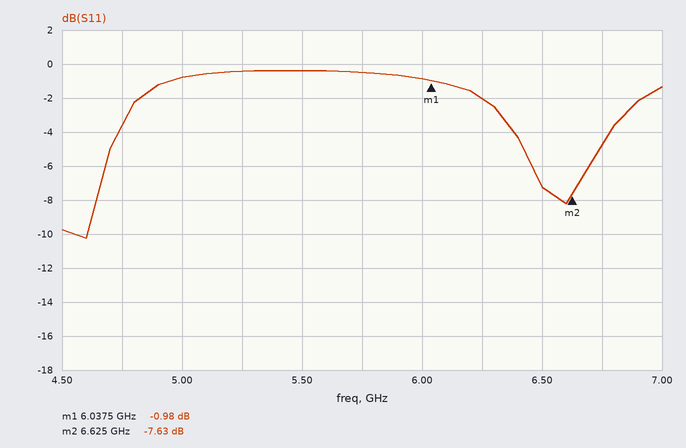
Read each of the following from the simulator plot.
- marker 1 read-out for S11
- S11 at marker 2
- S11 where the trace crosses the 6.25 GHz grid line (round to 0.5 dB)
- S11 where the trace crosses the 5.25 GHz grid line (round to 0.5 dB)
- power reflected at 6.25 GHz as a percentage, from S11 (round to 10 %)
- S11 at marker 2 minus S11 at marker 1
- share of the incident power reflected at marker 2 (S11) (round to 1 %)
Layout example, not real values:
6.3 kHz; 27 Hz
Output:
-0.98 dB; -7.63 dB; -2.0 dB; -0.5 dB; 60 %; -6.65 dB; 17 %
